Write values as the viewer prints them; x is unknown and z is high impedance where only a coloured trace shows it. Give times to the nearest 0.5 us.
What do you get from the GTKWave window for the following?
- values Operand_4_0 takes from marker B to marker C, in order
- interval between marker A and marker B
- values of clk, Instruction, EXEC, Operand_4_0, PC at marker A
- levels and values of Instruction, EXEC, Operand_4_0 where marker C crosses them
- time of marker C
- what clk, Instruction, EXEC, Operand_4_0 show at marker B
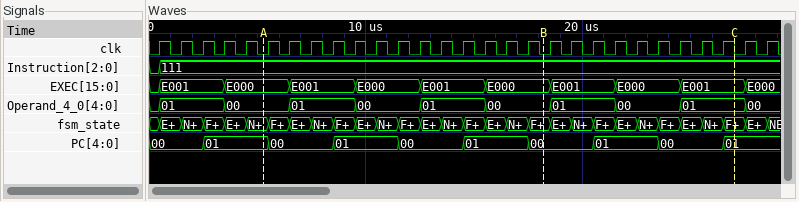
00, 01, 00, 01
13 us
clk=0, Instruction=111, EXEC=E000, Operand_4_0=00, PC=01
Instruction=111, EXEC=E001, Operand_4_0=01
27 us
clk=0, Instruction=111, EXEC=E000, Operand_4_0=00
